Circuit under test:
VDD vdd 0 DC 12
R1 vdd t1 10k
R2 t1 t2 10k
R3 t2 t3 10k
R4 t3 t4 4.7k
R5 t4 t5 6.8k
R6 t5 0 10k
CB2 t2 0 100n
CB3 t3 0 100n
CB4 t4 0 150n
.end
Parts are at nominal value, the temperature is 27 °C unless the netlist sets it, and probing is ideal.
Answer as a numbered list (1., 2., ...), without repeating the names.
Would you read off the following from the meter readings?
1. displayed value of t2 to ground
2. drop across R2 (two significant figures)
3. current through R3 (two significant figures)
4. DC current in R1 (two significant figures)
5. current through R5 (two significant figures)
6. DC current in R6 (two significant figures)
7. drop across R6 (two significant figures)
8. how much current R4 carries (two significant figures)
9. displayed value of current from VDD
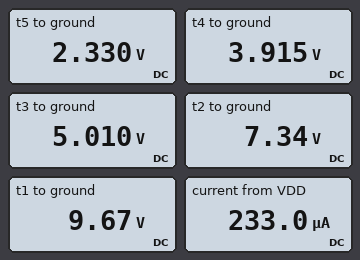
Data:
1. 7.34 V
2. 2.3 V
3. 230 µA
4. 230 µA
5. 230 µA
6. 230 µA
7. 2.3 V
8. 230 µA
9. 233.0 µA
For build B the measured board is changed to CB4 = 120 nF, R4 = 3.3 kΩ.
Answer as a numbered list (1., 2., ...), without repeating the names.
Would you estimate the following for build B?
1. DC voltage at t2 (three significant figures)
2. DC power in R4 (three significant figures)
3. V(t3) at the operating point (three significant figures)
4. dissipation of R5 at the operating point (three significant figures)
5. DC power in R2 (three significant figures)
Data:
1. 7.21 V
2. 189 µW
3. 4.81 V
4. 390 µW
5. 574 µW
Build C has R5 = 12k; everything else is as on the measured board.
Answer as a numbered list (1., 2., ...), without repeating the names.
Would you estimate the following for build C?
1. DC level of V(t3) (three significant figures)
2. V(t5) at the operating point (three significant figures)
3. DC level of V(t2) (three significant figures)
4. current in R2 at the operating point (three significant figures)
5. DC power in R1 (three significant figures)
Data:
1. 5.65 V
2. 2.12 V
3. 7.77 V
4. 212 µA
5. 448 µW
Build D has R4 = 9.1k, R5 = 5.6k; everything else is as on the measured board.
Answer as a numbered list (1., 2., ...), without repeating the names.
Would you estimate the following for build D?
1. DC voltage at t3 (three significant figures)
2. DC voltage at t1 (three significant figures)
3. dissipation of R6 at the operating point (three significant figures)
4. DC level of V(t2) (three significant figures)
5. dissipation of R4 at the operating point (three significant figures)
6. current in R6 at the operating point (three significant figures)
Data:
1. 5.42 V
2. 9.81 V
3. 481 µW
4. 7.61 V
5. 438 µW
6. 219 µA
